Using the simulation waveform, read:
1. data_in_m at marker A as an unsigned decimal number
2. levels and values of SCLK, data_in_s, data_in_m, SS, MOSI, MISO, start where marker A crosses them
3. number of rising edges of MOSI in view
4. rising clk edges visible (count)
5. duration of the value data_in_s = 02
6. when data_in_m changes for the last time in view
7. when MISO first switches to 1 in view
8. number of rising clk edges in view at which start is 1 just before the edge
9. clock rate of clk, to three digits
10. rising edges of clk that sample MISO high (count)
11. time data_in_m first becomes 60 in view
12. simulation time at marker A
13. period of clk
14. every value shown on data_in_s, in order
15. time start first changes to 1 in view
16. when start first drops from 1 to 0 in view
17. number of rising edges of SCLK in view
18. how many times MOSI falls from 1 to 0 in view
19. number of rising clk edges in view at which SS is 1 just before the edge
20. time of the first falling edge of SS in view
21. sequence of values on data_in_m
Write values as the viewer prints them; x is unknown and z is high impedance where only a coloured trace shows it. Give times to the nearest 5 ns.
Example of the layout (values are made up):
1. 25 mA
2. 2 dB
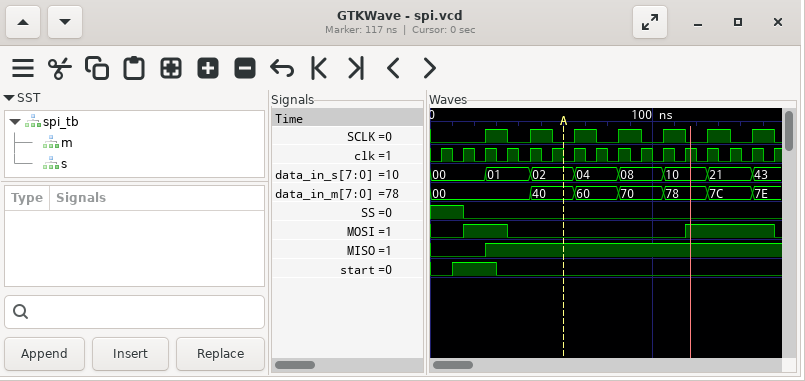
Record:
1. 64
2. SCLK=0, data_in_s=02, data_in_m=40, SS=0, MOSI=0, MISO=1, start=0
3. 2
4. 16
5. 20 ns
6. 145 ns
7. 25 ns
8. 2
9. 100 MHz
10. 13
11. 65 ns
12. 60 ns
13. 10 ns
14. 00, 01, 02, 04, 08, 10, 21, 43
15. 10 ns
16. 30 ns
17. 7
18. 2
19. 2
20. 15 ns
21. 00, 40, 60, 70, 78, 7C, 7E
